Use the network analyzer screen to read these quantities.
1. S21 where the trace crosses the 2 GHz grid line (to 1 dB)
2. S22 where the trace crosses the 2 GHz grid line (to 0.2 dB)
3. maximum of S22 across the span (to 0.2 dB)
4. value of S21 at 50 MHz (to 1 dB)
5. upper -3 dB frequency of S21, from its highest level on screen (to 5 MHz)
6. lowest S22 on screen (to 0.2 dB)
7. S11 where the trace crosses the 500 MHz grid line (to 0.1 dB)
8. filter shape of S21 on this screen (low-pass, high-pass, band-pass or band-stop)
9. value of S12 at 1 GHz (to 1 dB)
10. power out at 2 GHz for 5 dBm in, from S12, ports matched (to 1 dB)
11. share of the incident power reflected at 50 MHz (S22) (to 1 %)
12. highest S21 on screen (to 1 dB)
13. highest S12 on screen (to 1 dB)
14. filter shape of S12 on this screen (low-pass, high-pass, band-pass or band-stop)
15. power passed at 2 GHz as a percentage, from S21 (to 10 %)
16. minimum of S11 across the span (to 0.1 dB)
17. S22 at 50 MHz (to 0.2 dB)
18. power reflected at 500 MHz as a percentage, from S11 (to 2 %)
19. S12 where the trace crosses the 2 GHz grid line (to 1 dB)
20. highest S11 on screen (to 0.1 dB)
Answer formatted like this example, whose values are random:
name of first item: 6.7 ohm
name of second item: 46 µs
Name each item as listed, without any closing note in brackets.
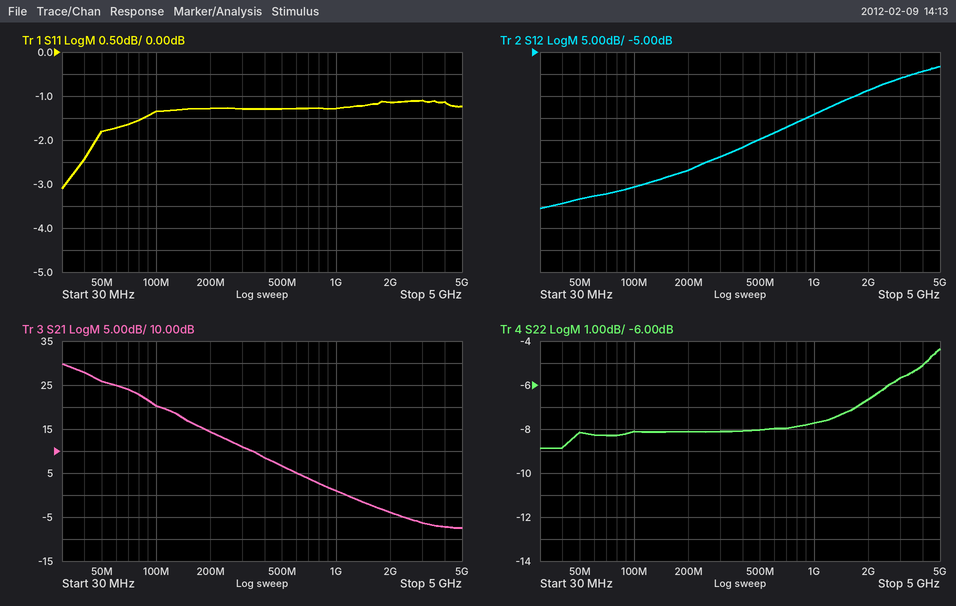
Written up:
S21 where the trace crosses the 2 GHz grid line: -4 dB
S22 where the trace crosses the 2 GHz grid line: -6.6 dB
maximum of S22 across the span: -4.4 dB
value of S21 at 50 MHz: 26 dB
upper -3 dB frequency of S21, from its highest level on screen: 45 MHz
lowest S22 on screen: -8.8 dB
S11 where the trace crosses the 500 MHz grid line: -1.3 dB
filter shape of S21 on this screen: low-pass
value of S12 at 1 GHz: -19 dB
power out at 2 GHz for 5 dBm in, from S12, ports matched: -9 dBm
share of the incident power reflected at 50 MHz (S22): 15 %
highest S21 on screen: 30 dB
highest S12 on screen: -8 dB
filter shape of S12 on this screen: high-pass
power passed at 2 GHz as a percentage, from S21: 40 %
minimum of S11 across the span: -3.1 dB
S22 at 50 MHz: -8.2 dB
power reflected at 500 MHz as a percentage, from S11: 74 %
S12 where the trace crosses the 2 GHz grid line: -14 dB
highest S11 on screen: -1.1 dB
